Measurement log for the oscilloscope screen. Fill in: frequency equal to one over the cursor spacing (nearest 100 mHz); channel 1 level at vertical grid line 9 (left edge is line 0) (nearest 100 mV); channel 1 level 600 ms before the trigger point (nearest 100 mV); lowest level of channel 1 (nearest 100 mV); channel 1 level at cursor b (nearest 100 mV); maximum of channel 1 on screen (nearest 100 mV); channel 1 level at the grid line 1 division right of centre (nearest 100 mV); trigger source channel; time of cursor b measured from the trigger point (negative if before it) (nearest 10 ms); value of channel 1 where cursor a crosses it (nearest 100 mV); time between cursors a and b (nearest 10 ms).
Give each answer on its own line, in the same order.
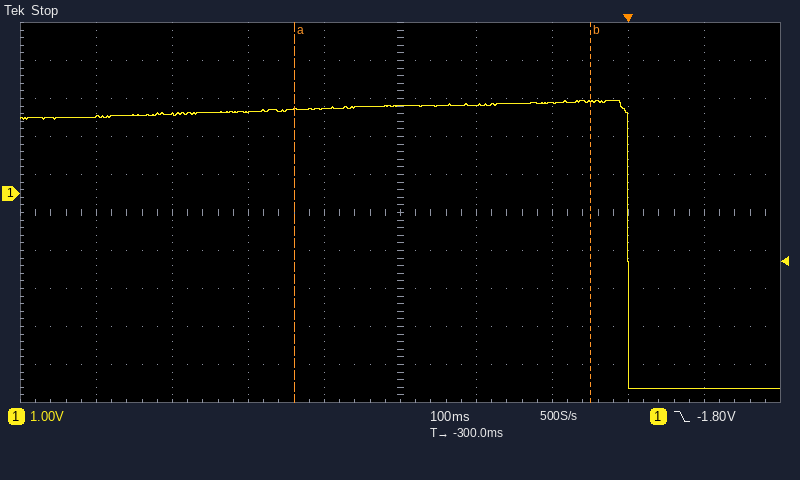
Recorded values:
2.6 Hz
-5.1 V
2.1 V
-5.1 V
2.4 V
2.4 V
2.3 V
channel 1
-50 ms
2.2 V
390 ms
